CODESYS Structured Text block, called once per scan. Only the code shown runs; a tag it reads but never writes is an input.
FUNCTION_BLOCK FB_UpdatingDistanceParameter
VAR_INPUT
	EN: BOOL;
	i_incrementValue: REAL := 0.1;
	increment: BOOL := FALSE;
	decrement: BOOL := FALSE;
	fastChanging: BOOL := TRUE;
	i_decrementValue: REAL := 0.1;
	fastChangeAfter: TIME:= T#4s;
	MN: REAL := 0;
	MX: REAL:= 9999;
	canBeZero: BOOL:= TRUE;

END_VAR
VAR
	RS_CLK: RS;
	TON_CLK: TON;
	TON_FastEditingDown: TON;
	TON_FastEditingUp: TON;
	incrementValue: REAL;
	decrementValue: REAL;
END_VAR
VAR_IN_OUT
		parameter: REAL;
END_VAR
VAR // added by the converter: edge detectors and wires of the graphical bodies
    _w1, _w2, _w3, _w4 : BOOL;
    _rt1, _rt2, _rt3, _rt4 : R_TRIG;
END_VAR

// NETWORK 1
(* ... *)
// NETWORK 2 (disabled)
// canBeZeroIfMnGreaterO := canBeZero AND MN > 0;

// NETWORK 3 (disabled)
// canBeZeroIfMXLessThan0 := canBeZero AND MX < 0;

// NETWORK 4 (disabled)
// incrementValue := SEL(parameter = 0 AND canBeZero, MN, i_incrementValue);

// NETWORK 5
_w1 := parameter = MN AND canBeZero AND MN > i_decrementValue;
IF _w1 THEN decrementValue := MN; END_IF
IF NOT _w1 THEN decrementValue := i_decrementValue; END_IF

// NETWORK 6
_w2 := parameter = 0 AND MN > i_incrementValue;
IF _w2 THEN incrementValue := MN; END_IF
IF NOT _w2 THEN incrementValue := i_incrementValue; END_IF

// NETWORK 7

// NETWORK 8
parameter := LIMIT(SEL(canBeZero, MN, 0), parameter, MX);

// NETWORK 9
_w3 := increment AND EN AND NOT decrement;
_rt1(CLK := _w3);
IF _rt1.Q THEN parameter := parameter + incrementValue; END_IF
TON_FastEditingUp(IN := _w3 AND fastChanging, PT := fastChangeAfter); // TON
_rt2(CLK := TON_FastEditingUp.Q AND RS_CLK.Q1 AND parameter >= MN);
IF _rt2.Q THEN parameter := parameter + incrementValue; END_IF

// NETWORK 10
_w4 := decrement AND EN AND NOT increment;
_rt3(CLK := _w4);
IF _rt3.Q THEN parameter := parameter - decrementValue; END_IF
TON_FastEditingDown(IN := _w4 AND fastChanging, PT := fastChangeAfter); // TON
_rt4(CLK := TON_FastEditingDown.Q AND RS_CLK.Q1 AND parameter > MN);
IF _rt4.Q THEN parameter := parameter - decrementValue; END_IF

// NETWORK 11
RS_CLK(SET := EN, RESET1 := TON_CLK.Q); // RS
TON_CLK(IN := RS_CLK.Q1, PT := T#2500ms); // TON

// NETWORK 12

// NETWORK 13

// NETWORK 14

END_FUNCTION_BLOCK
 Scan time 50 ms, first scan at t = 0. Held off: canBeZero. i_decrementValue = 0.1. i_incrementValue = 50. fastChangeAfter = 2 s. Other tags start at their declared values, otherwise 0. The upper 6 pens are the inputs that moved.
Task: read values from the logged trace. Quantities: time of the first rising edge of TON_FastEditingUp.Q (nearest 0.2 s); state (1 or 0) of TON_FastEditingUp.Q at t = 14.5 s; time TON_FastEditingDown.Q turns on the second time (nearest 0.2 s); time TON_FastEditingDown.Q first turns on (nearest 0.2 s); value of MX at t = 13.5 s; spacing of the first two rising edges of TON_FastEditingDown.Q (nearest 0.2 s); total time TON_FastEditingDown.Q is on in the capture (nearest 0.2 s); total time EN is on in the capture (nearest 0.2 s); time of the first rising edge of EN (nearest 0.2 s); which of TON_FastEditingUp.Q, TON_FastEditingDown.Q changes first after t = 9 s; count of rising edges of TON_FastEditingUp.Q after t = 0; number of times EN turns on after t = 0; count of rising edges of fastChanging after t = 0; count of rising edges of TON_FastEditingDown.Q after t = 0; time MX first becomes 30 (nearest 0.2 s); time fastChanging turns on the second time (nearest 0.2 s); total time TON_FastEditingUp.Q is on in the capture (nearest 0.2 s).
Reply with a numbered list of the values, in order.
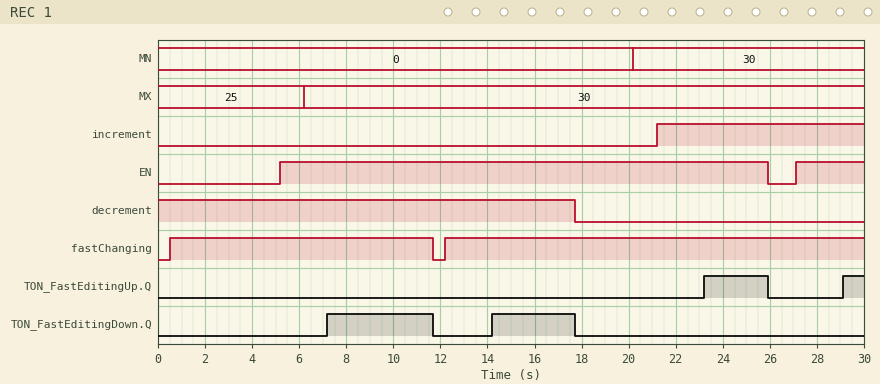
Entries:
1. 23.2 s
2. 0
3. 14.2 s
4. 7.2 s
5. 30
6. 7.0 s
7. 8.0 s
8. 23.6 s
9. 5.2 s
10. TON_FastEditingDown.Q
11. 2
12. 2
13. 2
14. 2
15. 6.2 s
16. 12.2 s
17. 3.6 s
